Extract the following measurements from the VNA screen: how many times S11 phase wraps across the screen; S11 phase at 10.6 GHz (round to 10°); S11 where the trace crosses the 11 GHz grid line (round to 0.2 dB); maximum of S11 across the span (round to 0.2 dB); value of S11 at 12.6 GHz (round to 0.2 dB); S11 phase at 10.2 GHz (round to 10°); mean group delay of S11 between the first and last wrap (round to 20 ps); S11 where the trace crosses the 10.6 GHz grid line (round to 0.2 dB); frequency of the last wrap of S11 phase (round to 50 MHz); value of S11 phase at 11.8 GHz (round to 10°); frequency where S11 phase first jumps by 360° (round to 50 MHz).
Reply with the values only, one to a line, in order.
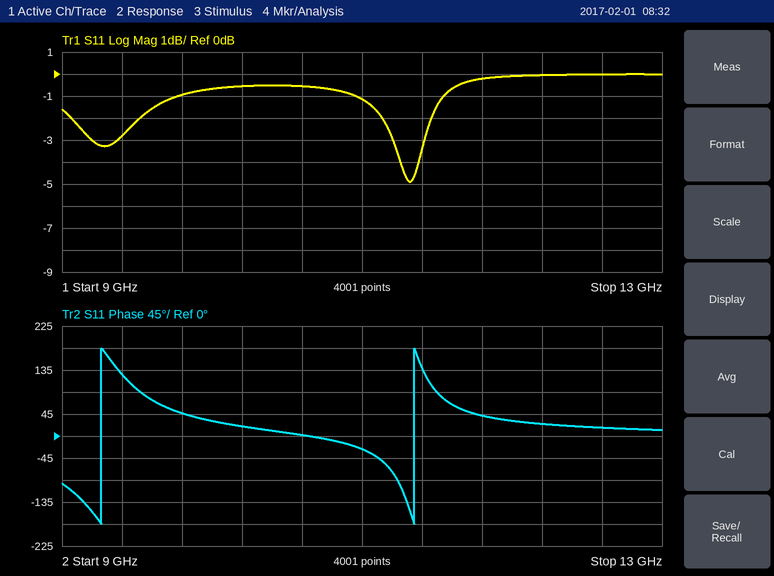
2
0°
-1.2 dB
0.0 dB
0.0 dB
20°
480 ps
-0.6 dB
11.35 GHz
40°
9.25 GHz
